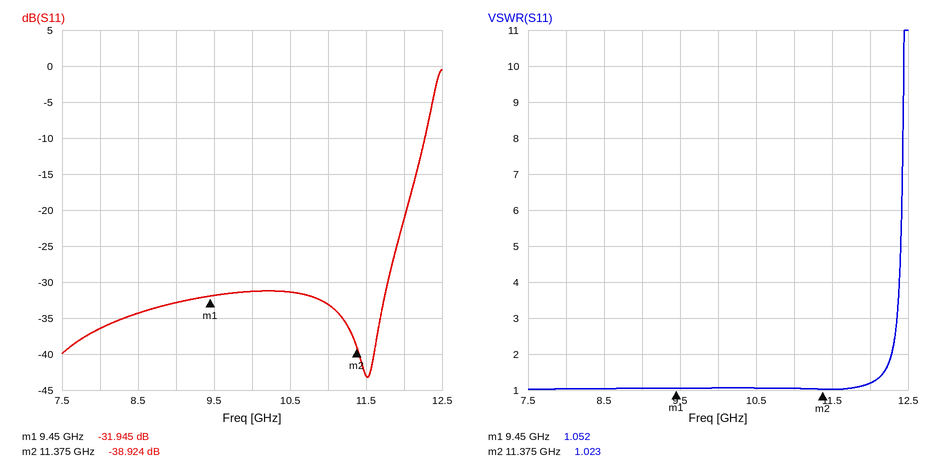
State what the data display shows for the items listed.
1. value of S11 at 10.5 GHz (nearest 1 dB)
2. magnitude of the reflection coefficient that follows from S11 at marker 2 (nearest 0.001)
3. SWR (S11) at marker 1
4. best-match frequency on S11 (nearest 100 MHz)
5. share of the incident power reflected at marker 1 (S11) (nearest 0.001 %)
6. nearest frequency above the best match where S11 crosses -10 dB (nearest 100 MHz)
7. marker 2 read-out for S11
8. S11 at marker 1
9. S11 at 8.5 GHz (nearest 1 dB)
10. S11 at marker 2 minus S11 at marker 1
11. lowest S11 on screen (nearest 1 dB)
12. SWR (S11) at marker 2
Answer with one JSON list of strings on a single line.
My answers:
["-31 dB", "0.011", "1.052", "11.5 GHz", "0.064 %", "12.3 GHz", "-38.924 dB", "-31.945 dB", "-34 dB", "-6.979 dB", "-43 dB", "1.023"]
